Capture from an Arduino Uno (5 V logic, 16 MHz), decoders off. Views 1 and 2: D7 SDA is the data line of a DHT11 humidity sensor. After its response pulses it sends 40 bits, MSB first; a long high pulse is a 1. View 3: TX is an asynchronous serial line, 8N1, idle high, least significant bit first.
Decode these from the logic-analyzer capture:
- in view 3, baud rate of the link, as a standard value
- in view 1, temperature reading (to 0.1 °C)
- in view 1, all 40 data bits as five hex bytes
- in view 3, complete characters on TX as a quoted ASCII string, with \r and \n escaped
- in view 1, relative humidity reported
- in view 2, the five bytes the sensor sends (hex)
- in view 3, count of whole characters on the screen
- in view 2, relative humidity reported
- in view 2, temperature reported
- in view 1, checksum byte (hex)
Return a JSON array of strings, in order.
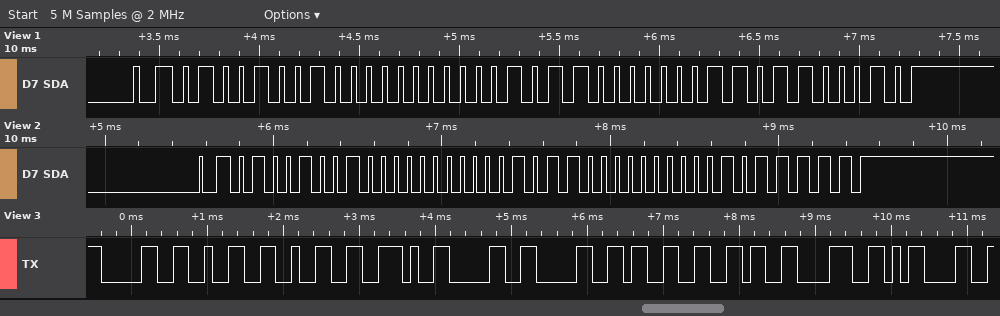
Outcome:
["9600 baud", "22.3 °C", "49 00 16 03 62", "\"022.00368\\r\"", "73 %", "49 00 16 00 5F", "10", "73 %", "22.0 °C", "0x62"]
